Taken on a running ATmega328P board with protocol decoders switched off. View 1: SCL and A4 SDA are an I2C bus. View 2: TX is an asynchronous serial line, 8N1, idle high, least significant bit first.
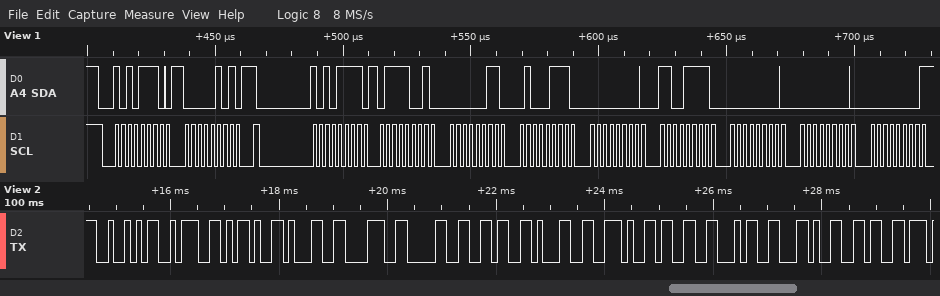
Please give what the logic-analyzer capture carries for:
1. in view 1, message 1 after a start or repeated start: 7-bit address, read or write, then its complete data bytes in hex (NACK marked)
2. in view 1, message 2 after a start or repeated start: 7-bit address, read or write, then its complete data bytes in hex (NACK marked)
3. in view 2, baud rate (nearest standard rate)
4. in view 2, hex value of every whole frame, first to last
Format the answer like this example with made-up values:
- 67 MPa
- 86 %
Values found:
- 0x57 write: 05
- 0x57 read: 79 03 47 00 CF 00 00 00 NACK
- 9600 baud
- 52 3A 2D 31 38 30 36 31 2E 33 34 2C 36
